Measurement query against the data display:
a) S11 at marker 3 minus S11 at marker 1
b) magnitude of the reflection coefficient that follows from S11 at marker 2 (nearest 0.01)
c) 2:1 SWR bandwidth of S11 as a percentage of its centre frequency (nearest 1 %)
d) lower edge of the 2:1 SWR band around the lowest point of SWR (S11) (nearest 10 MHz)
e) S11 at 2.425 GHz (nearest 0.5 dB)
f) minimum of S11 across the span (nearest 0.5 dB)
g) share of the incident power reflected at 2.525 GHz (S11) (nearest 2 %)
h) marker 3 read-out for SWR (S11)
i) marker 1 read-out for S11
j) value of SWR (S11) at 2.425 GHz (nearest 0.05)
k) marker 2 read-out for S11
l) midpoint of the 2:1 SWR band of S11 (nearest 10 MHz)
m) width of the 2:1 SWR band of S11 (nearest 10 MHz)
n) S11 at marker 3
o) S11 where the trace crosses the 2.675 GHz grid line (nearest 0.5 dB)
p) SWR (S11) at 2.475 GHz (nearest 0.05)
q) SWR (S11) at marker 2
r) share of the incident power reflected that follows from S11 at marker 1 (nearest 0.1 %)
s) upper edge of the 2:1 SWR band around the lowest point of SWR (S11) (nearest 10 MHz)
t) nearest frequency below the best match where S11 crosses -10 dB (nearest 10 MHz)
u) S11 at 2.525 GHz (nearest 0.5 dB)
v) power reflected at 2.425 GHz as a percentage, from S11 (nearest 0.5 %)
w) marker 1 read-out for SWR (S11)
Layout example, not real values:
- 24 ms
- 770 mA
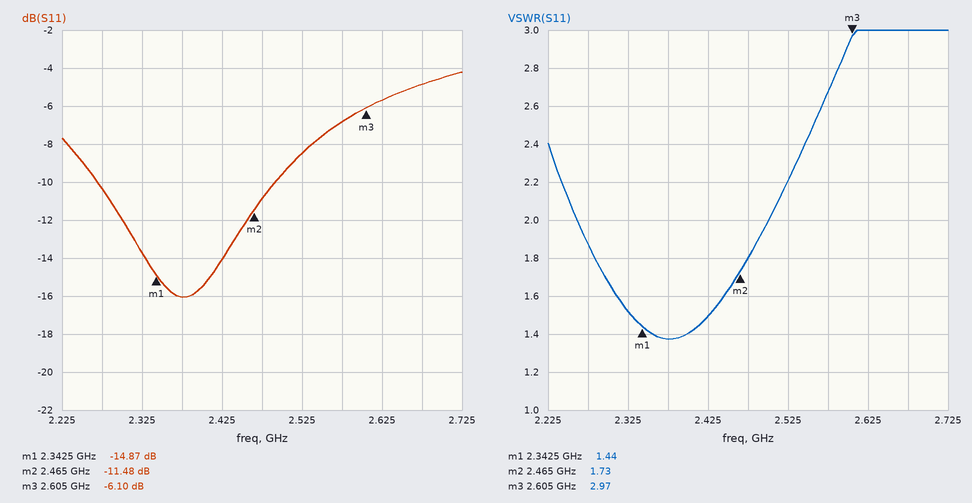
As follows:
- 8.77 dB
- 0.27
- 10 %
- 2.26 GHz
- -14.0 dB
- -16.0 dB
- 14 %
- 2.97
- -14.87 dB
- 1.50
- -11.48 dB
- 2.38 GHz
- 240 MHz
- -6.10 dB
- -5.0 dB
- 1.80
- 1.73
- 3.3 %
- 2.50 GHz
- 2.27 GHz
- -8.5 dB
- 4.0 %
- 1.44
